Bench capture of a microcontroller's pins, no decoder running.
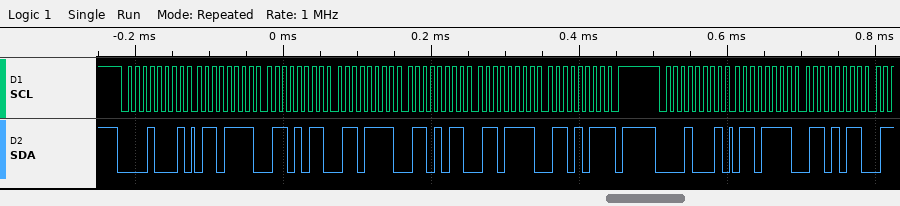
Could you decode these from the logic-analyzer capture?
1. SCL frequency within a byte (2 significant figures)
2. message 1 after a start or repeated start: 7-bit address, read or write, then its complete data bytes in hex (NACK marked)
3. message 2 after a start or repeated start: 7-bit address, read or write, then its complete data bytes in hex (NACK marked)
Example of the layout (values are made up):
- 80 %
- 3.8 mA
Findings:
- 100 kHz
- 0x08 read: 6F 6B 6F 6B 6F 6B NACK
- 0x08 read: 6F 6B
